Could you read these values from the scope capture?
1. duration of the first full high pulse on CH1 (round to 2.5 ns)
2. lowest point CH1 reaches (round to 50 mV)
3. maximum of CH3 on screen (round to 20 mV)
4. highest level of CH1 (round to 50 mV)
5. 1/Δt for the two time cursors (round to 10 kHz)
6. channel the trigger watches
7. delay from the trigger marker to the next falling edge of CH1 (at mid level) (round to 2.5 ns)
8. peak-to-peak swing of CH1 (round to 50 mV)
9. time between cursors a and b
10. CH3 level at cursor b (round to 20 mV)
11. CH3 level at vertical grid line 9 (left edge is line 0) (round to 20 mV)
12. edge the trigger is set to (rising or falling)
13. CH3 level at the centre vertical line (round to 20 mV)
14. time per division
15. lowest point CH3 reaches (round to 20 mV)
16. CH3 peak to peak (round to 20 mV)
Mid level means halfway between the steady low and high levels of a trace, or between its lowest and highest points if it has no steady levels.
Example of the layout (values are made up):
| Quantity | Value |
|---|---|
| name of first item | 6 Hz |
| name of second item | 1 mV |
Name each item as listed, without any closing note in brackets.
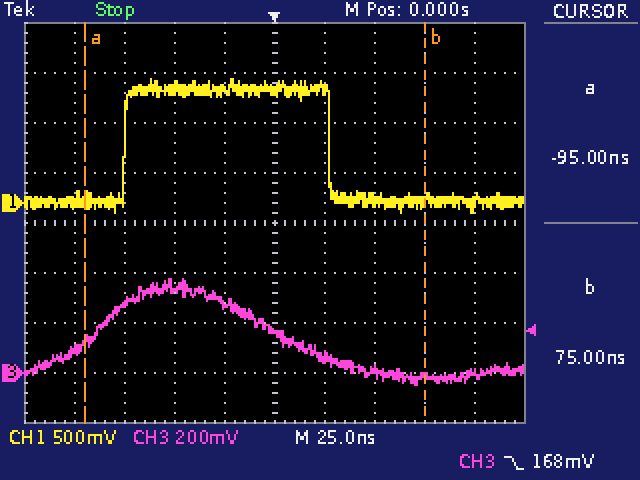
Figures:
| Quantity | Value |
|---|---|
| duration of the first full high pulse on CH1 | 102.5 ns |
| lowest point CH1 reaches | -100 mV |
| maximum of CH3 on screen | 380 mV |
| highest level of CH1 | 1.25 V |
| 1/Δt for the two time cursors | 5.88 MHz |
| channel the trigger watches | CH3 |
| delay from the trigger marker to the next falling edge of CH1 (at mid level) | 27.5 ns |
| peak-to-peak swing of CH1 | 1.35 V |
| time between cursors a and b | 170.0 ns |
| CH3 level at cursor b | -20 mV |
| CH3 level at vertical grid line 9 (left edge is line 0) | 0 mV |
| edge the trigger is set to | falling |
| CH3 level at the centre vertical line | 160 mV |
| time per division | 25 ns |
| lowest point CH3 reaches | -40 mV |
| CH3 peak to peak | 420 mV |
